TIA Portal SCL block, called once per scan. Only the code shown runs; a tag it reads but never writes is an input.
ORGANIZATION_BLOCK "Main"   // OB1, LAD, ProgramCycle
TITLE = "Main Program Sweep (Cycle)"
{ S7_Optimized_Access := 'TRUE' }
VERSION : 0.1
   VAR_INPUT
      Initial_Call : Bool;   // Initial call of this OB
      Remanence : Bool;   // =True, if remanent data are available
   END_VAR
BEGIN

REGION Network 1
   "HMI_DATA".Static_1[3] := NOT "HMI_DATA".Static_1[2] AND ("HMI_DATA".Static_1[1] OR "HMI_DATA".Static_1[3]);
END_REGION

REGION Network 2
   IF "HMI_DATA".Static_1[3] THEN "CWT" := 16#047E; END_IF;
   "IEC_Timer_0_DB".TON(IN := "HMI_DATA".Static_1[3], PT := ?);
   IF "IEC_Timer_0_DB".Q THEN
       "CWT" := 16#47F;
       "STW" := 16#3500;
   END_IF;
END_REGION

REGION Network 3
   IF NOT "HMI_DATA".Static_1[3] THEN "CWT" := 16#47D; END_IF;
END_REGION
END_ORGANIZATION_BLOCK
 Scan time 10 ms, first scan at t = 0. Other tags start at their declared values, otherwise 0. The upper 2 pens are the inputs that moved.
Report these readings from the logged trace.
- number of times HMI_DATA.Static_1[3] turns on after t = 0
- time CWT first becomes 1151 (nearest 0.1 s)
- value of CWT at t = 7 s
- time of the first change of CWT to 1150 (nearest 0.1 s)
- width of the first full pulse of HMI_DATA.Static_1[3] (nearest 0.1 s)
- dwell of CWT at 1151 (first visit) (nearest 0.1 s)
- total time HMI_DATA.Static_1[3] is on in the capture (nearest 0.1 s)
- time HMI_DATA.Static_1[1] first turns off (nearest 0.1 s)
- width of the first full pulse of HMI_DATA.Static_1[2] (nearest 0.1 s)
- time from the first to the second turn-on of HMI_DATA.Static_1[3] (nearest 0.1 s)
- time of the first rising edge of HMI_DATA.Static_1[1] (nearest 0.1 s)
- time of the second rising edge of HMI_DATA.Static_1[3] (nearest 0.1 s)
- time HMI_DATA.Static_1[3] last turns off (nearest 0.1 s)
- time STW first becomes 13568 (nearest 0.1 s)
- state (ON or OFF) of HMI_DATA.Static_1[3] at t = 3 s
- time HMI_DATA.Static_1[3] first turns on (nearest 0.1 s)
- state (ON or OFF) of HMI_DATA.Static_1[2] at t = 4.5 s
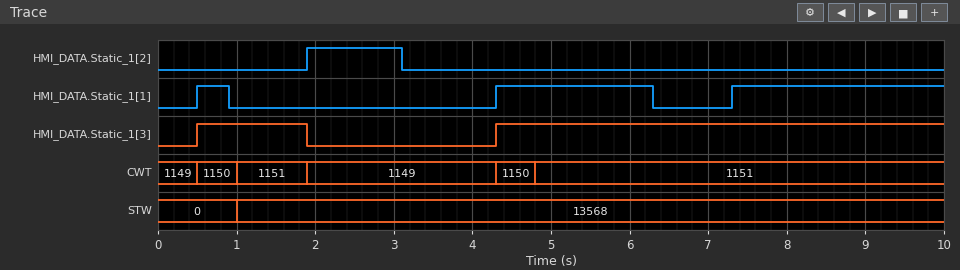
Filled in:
2
1.0 s
1151
0.5 s
1.4 s
0.9 s
7.1 s
0.9 s
1.2 s
3.8 s
0.5 s
4.3 s
1.9 s
1.0 s
OFF
0.5 s
OFF
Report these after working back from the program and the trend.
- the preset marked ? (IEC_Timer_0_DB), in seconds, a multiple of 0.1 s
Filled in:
0.5 s
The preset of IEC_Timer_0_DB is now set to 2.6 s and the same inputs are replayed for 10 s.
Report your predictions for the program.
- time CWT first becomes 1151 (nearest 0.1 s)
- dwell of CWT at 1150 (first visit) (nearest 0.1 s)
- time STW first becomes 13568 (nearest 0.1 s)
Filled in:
6.9 s
1.4 s
6.9 s
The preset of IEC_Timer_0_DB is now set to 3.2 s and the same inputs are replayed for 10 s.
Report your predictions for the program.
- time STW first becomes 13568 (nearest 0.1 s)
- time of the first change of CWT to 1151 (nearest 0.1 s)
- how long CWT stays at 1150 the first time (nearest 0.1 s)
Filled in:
7.5 s
7.5 s
1.4 s
